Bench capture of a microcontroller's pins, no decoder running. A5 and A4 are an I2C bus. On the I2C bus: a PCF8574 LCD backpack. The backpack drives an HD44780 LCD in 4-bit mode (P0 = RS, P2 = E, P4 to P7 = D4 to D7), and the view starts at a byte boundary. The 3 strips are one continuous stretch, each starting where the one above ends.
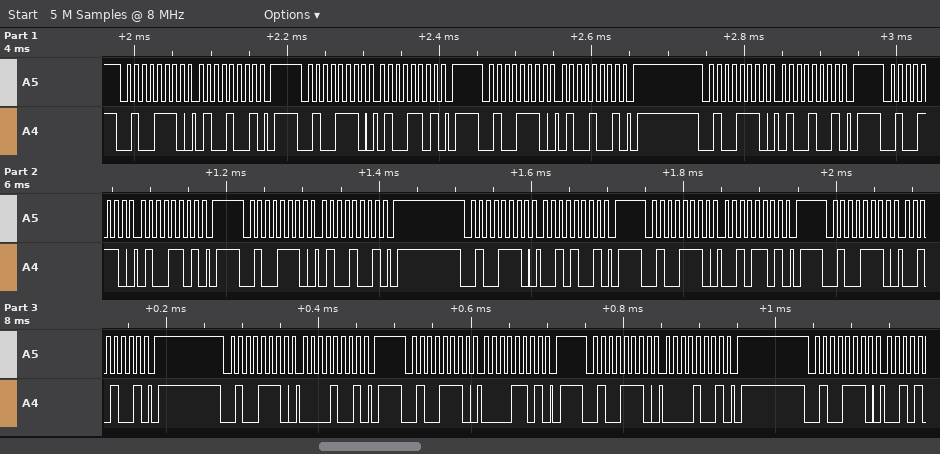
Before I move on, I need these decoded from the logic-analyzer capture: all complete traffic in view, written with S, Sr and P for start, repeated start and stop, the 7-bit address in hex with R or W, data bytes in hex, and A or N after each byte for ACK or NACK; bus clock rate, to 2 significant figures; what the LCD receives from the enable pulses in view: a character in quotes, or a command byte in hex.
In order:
S 27W A 49 A P S 27W A 4D A P S 27W A 49 A P S 27W A 49 A P S 27W A 4D A P S 27W A 49 A P S 27W A 29 A P S 27W A 2D A P S 27W A 29 A P S 27W A 09 A P S 27W A 0D A P S 27W A 09 A P S 27W A
100 kHz
'D' ' '
